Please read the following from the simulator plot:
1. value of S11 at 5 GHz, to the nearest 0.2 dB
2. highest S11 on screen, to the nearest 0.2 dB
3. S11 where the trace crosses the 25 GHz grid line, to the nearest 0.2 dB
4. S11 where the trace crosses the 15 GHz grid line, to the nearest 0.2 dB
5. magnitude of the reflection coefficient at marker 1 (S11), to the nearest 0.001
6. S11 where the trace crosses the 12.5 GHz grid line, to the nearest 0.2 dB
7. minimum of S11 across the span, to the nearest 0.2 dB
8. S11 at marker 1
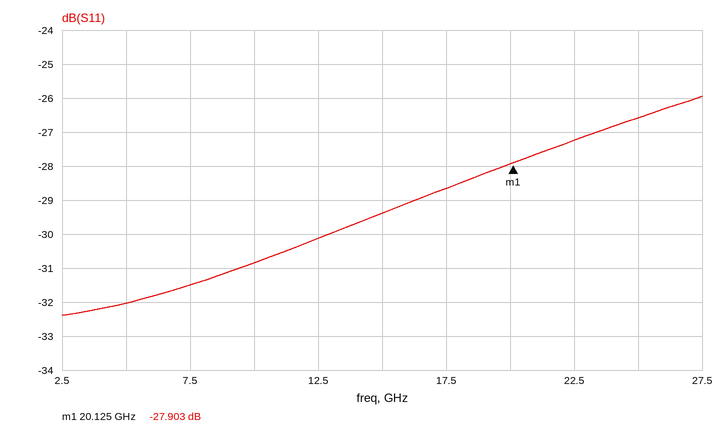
-32.0 dB
-26.0 dB
-26.6 dB
-29.4 dB
0.040
-30.2 dB
-32.4 dB
-27.903 dB
